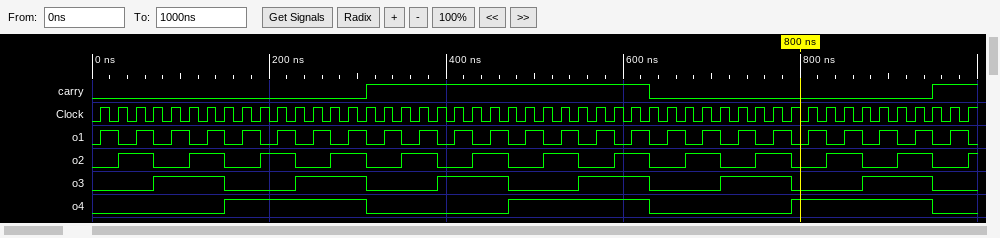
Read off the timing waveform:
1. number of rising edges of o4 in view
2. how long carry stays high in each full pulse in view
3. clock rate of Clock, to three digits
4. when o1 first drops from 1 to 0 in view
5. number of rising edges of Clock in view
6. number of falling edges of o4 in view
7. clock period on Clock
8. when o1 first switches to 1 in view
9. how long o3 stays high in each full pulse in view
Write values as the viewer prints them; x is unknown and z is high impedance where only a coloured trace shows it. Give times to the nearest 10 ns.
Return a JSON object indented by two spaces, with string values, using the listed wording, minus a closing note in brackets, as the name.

{
  "number of rising edges of o4 in view": "3",
  "how long carry stays high in each full pulse in view": "320 ns",
  "clock rate of Clock, to three digits": "50.0 MHz",
  "when o1 first drops from 1 to 0 in view": "30 ns",
  "number of rising edges of Clock in view": "50",
  "number of falling edges of o4 in view": "3",
  "clock period on Clock": "20 ns",
  "when o1 first switches to 1 in view": "10 ns",
  "how long o3 stays high in each full pulse in view": "80 ns, 80 ns, 80 ns, 80 ns, 80 ns, 80 ns"
}
